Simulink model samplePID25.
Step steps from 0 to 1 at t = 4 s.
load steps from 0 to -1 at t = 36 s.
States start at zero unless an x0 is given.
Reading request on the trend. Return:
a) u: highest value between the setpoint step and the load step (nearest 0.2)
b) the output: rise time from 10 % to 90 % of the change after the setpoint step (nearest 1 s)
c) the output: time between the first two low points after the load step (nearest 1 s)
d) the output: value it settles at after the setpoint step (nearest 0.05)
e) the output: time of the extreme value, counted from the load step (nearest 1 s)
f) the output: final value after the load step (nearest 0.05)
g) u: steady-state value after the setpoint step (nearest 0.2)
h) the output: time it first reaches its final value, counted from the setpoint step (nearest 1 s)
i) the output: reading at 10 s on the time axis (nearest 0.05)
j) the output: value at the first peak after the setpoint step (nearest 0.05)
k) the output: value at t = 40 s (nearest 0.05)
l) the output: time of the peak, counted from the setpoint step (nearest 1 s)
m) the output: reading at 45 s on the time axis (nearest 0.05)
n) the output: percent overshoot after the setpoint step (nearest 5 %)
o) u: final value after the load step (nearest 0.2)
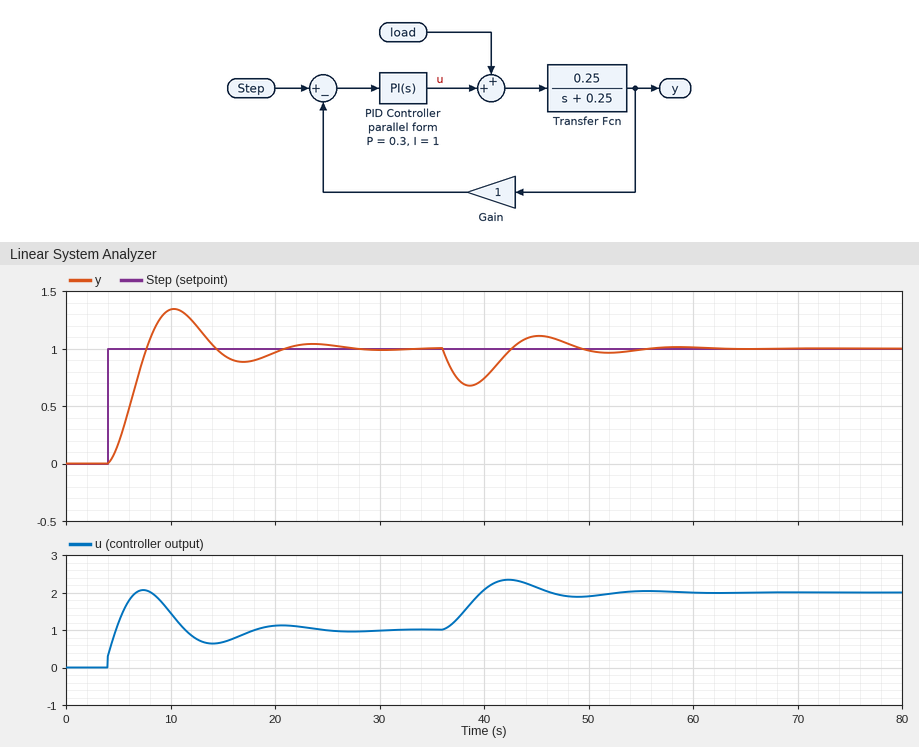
2.0
3 s
13 s
1.00
3 s
1.00
1.0
4 s
1.35
1.35
0.75
6 s
1.10
35 %
2.0
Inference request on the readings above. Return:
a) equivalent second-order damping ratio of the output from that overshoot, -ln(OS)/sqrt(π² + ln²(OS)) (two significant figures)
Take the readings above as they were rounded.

0.32
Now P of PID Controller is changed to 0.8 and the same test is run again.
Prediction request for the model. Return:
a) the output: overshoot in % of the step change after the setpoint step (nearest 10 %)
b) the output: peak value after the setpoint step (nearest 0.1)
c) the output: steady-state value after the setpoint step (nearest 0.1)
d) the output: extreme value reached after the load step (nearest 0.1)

20 %
1.2
1.0
0.7
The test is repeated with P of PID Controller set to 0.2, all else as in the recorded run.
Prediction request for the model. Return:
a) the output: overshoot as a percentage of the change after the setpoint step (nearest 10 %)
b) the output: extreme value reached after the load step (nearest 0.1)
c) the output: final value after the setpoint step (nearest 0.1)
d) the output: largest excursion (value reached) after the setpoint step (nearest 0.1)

40 %
0.7
1.0
1.4
